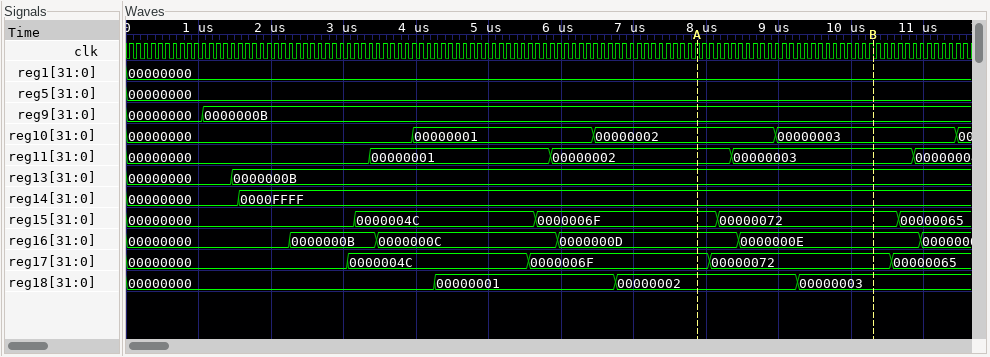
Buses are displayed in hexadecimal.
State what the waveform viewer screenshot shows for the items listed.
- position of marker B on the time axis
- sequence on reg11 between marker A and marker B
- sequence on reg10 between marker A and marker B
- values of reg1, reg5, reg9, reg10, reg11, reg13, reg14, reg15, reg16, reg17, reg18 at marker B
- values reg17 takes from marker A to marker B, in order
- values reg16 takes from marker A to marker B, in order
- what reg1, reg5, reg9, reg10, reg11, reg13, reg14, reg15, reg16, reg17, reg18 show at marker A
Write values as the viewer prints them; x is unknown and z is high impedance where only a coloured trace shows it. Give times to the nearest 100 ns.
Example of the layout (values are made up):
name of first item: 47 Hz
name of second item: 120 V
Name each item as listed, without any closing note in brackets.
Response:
position of marker B on the time axis: 10300 ns
sequence on reg11 between marker A and marker B: 00000002, 00000003
sequence on reg10 between marker A and marker B: 00000002, 00000003
values of reg1, reg5, reg9, reg10, reg11, reg13, reg14, reg15, reg16, reg17, reg18 at marker B: reg1=00000000, reg5=00000000, reg9=0000000B, reg10=00000003, reg11=00000003, reg13=0000000B, reg14=0000FFFF, reg15=00000072, reg16=0000000E, reg17=00000072, reg18=00000003
values reg17 takes from marker A to marker B, in order: 0000006F, 00000072
values reg16 takes from marker A to marker B, in order: 0000000D, 0000000E
what reg1, reg5, reg9, reg10, reg11, reg13, reg14, reg15, reg16, reg17, reg18 show at marker A: reg1=00000000, reg5=00000000, reg9=0000000B, reg10=00000002, reg11=00000002, reg13=0000000B, reg14=0000FFFF, reg15=0000006F, reg16=0000000D, reg17=0000006F, reg18=00000002
